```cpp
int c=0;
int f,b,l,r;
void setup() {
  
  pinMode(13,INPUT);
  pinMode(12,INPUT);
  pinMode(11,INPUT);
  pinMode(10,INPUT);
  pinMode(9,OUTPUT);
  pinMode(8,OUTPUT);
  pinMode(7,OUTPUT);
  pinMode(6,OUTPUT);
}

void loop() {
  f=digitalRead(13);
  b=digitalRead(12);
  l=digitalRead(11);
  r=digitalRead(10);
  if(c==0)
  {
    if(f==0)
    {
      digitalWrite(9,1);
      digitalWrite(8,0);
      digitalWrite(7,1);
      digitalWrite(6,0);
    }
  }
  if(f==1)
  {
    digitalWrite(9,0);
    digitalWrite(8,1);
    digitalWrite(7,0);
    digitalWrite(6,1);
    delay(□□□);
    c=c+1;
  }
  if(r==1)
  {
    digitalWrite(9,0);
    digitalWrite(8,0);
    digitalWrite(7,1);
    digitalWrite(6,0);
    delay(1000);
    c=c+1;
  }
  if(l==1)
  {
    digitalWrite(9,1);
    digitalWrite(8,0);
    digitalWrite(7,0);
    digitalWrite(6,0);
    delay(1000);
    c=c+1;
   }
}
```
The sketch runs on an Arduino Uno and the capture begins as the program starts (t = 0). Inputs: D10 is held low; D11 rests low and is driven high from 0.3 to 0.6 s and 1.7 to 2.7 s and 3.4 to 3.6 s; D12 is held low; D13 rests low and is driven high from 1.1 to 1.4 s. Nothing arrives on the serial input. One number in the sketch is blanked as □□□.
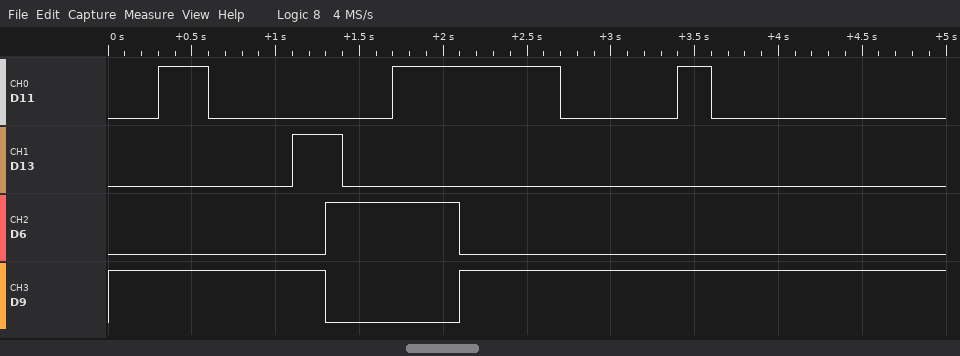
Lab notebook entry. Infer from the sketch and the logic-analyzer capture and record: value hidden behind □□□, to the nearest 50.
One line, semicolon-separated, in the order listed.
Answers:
800
